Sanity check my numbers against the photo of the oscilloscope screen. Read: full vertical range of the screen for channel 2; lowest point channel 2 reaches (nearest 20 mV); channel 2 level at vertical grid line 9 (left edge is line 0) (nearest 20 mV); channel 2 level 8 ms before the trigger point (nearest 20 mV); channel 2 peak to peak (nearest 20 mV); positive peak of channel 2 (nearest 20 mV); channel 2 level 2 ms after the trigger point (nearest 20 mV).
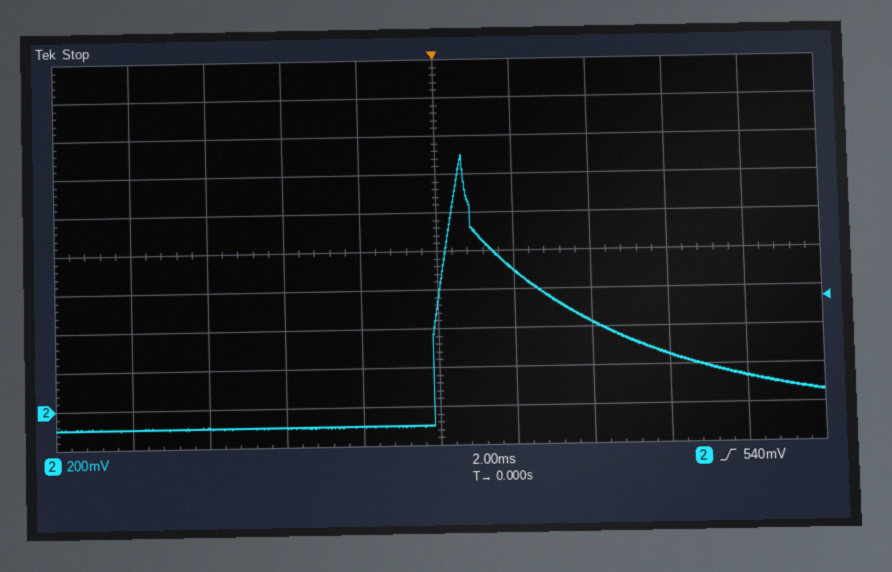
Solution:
2 V
-100 mV
140 mV
-100 mV
1.40 V
1.30 V
700 mV
